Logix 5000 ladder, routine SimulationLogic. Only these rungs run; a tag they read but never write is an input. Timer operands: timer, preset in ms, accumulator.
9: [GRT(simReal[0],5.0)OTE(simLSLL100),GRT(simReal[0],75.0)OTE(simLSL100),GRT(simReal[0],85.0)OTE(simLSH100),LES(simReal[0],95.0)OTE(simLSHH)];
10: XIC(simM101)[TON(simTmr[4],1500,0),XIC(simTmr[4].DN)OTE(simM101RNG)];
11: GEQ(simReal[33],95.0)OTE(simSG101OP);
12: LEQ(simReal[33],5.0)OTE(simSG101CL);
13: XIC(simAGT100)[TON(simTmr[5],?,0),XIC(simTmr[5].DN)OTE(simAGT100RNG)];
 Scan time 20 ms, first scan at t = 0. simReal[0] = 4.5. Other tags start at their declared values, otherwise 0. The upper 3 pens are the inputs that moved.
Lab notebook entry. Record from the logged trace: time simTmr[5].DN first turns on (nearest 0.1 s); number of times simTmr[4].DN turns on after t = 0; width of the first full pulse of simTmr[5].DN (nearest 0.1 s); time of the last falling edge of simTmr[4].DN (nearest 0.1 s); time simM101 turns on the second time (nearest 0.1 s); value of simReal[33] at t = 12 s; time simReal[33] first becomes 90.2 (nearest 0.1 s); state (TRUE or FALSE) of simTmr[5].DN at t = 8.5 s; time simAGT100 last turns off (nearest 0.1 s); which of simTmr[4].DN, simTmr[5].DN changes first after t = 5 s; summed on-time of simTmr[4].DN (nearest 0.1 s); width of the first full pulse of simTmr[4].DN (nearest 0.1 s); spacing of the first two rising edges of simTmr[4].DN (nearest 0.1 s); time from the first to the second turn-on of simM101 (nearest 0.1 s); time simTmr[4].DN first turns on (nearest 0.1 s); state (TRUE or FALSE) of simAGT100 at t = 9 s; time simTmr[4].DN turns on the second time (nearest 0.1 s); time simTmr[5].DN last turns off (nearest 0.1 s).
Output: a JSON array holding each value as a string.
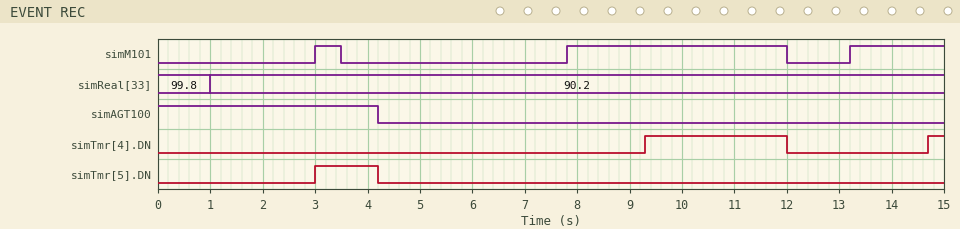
["3.0 s", "2", "1.2 s", "12.0 s", "7.8 s", "90.2", "1.0 s", "FALSE", "4.2 s", "simTmr[4].DN", "3.0 s", "2.7 s", "5.4 s", "4.8 s", "9.3 s", "FALSE", "14.7 s", "4.2 s"]
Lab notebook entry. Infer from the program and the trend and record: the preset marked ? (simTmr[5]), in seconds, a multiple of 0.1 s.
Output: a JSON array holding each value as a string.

["3.0 s"]
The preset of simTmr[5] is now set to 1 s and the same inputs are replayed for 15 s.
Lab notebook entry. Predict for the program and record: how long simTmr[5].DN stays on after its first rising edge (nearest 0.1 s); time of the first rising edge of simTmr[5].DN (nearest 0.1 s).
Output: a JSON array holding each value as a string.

["3.2 s", "1.0 s"]
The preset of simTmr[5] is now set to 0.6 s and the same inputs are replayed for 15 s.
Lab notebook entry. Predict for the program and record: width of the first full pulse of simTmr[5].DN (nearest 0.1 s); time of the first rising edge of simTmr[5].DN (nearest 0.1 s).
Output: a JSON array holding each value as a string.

["3.6 s", "0.6 s"]
